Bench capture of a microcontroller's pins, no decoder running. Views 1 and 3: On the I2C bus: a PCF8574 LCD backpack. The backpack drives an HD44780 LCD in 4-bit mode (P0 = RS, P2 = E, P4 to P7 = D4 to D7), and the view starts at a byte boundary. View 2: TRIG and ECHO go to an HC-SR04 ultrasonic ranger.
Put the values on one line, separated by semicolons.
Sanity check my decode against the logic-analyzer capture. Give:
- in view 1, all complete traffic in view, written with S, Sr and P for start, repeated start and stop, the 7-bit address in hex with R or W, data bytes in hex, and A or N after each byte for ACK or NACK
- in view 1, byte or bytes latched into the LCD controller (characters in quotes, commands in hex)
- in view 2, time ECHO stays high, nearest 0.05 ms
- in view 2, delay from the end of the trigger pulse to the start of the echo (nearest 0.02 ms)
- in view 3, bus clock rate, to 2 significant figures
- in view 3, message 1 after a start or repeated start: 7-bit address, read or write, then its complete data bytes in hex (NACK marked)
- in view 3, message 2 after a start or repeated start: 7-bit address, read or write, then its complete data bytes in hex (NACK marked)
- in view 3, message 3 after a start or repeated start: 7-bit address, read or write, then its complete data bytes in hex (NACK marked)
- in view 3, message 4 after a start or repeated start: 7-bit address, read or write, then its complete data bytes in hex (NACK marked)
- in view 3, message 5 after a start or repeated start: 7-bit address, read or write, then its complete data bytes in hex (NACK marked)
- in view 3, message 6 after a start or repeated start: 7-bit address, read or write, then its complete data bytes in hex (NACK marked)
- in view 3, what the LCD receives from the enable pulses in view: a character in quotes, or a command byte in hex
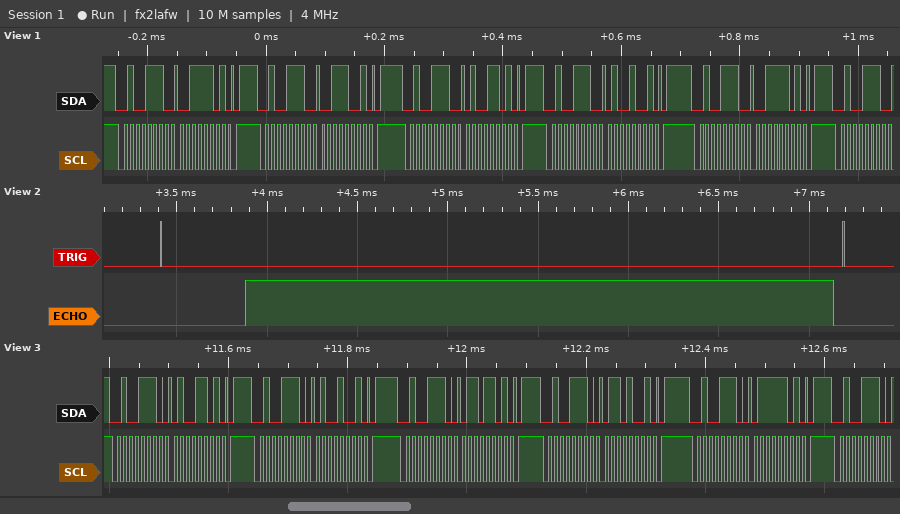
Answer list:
S 27W A 3D A P S 27W A 39 A P S 27W A 4D A P S 27W A 49 A P S 27W A 3D A P S 27W A; '4'; 3.25 ms; 0.46 ms; 100 kHz; 0x27 write: 4D; 0x27 write: 49; 0x27 write: 6D; 0x27 write: 69; 0x27 write: 7D; 0x27 write; 'F'
